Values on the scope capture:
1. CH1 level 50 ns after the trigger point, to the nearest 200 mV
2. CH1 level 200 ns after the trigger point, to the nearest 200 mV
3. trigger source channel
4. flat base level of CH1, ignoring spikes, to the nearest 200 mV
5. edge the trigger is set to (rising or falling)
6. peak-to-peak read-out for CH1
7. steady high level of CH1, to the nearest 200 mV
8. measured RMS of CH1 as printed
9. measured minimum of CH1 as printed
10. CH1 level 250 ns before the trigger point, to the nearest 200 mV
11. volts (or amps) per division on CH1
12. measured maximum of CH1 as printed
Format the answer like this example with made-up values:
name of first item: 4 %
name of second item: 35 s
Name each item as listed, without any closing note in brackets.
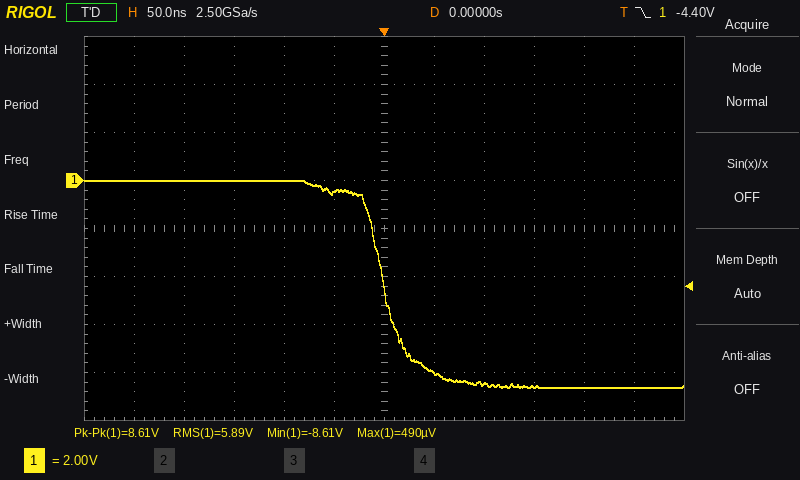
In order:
CH1 level 50 ns after the trigger point, to the nearest 200 mV: -8.0 V
CH1 level 200 ns after the trigger point, to the nearest 200 mV: -8.6 V
trigger source channel: CH1
flat base level of CH1, ignoring spikes, to the nearest 200 mV: -8.6 V
edge the trigger is set to: falling
peak-to-peak read-out for CH1: 8.61 V
steady high level of CH1, to the nearest 200 mV: 0.0 V
measured RMS of CH1 as printed: 5.89 V
measured minimum of CH1 as printed: -8.61 V
CH1 level 250 ns before the trigger point, to the nearest 200 mV: 0.0 V
volts (or amps) per division on CH1: 2 V
measured maximum of CH1 as printed: 490 µV
